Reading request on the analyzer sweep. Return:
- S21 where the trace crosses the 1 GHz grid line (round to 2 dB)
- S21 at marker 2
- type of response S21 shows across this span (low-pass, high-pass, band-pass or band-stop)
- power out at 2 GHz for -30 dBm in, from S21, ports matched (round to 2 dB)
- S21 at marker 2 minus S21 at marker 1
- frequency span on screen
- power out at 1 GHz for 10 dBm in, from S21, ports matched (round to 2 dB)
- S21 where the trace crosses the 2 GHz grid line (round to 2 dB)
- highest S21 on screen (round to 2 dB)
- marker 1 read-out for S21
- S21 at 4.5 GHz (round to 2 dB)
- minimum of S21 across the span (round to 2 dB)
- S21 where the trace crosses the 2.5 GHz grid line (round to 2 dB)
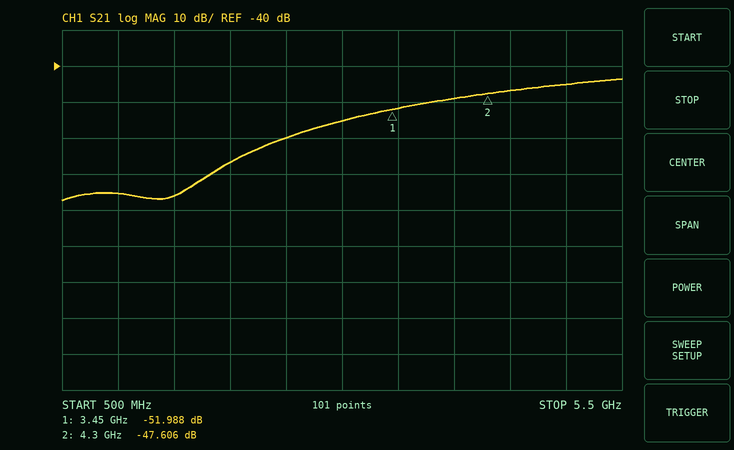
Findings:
-76 dB
-47.606 dB
high-pass
-96 dBm
4.382 dB
5 GHz
-66 dBm
-66 dB
-44 dB
-51.988 dB
-46 dB
-78 dB
-60 dB
